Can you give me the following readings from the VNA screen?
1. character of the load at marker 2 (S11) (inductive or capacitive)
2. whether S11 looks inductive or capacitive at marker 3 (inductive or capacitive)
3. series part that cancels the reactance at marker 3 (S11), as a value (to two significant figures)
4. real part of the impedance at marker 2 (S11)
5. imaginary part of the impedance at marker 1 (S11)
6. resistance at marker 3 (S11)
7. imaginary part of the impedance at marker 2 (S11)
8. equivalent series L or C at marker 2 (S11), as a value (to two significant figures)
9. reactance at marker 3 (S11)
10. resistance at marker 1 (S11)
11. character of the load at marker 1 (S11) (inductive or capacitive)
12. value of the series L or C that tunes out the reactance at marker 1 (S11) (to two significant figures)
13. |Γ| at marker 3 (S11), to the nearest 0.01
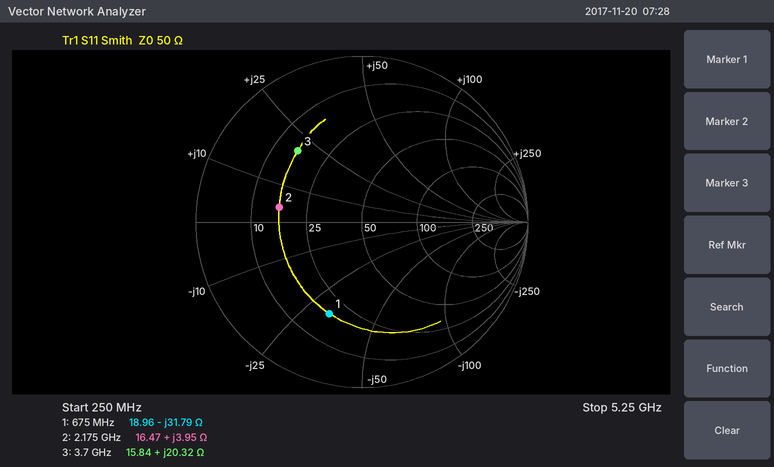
inductive
inductive
2.1 pF
16.47 Ω
-31.79 Ω
15.84 Ω
+3.95 Ω
290 pH
+20.32 Ω
18.96 Ω
capacitive
7.5 nH
0.58
